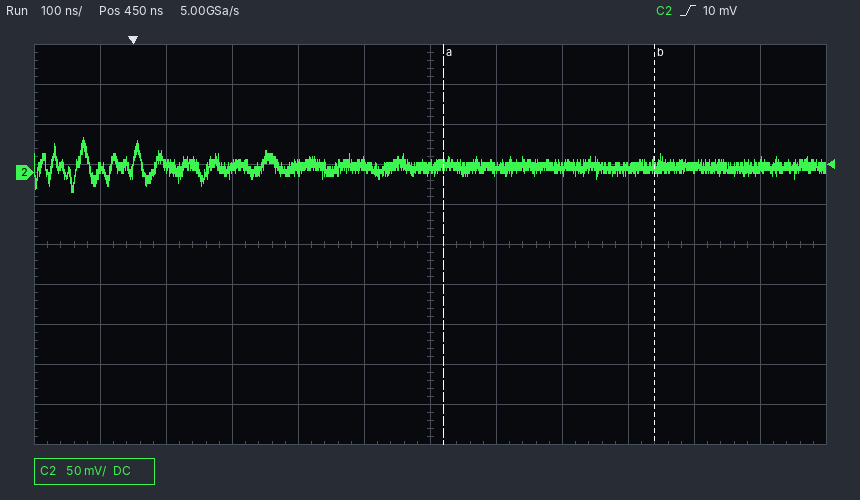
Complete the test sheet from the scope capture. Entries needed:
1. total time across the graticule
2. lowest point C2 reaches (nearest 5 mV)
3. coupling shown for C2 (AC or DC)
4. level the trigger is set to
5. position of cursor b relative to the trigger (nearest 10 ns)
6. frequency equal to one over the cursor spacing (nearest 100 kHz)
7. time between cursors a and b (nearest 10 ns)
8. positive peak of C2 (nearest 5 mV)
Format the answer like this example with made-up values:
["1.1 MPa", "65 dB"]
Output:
["1.2 µs", "-25 mV", "DC", "10 mV", "+790 ns", "3.1 MHz", "320 ns", "45 mV"]
